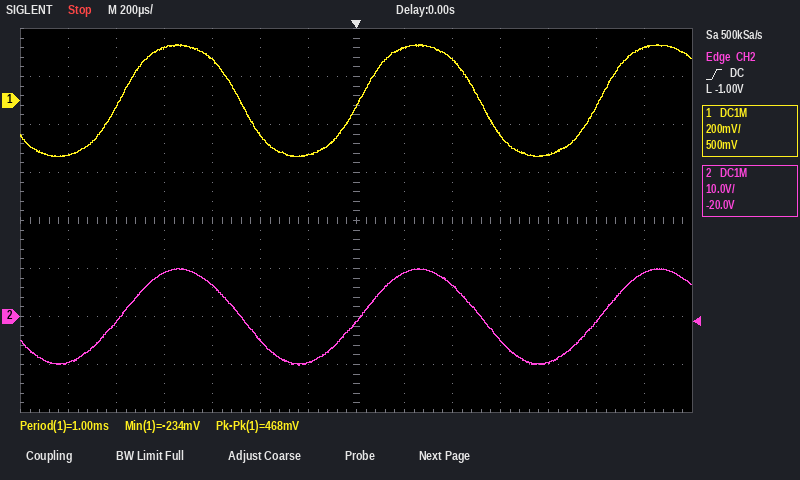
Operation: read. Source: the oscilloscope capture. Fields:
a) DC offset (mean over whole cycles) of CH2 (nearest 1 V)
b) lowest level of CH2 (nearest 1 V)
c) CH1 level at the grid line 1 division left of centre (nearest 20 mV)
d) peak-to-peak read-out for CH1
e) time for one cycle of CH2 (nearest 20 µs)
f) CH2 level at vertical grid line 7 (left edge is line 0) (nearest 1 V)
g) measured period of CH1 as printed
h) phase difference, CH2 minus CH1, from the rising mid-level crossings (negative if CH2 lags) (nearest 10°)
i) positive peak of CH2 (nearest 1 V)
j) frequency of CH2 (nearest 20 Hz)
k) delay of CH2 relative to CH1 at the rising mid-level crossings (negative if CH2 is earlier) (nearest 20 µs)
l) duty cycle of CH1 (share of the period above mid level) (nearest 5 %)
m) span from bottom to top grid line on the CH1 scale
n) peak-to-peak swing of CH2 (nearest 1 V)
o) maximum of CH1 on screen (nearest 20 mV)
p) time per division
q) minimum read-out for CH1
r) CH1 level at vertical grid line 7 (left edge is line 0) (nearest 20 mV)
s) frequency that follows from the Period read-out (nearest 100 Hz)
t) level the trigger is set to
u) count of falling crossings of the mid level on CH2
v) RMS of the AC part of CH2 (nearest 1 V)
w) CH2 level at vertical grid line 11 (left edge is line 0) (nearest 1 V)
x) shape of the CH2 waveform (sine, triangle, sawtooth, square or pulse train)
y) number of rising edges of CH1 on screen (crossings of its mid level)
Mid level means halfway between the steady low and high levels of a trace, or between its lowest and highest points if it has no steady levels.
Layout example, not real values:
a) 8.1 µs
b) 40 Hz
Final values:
a) 0 V
b) -10 V
c) -220 mV
d) 468 mV
e) 1.00 ms
f) -1 V
g) 1.00 ms
h) 0°
i) 10 V
j) 1.00 kHz
k) 0 µs
l) 50 %
m) 1.6 V
n) 20 V
o) 240 mV
p) 200 µs
q) -234 mV
r) -20 mV
s) 1.0 kHz
t) -1.00 V
u) 2
v) 7 V
w) -10 V
x) sine
y) 3
